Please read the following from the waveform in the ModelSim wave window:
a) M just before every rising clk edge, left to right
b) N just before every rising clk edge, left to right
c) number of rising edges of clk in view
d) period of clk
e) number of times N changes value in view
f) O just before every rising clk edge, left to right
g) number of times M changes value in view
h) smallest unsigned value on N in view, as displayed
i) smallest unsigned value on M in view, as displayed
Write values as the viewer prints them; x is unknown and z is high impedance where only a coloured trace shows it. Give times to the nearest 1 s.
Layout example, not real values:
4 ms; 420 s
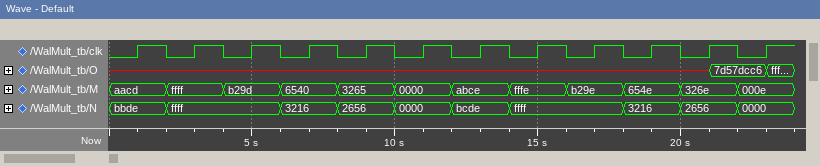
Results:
aacd, ffff, b29d, 6540, 3265, 0000, abce, fffe, b29e, 654e, 326e, 000e; bbde, ffff, ffff, 3216, 2656, 0000, bcde, ffff, ffff, 3216, 2656, 0000; 12; 2 s; 9; x, x, x, x, x, x, x, x, x, x, x, 7d57dcc6; 11; 0000; 0000
